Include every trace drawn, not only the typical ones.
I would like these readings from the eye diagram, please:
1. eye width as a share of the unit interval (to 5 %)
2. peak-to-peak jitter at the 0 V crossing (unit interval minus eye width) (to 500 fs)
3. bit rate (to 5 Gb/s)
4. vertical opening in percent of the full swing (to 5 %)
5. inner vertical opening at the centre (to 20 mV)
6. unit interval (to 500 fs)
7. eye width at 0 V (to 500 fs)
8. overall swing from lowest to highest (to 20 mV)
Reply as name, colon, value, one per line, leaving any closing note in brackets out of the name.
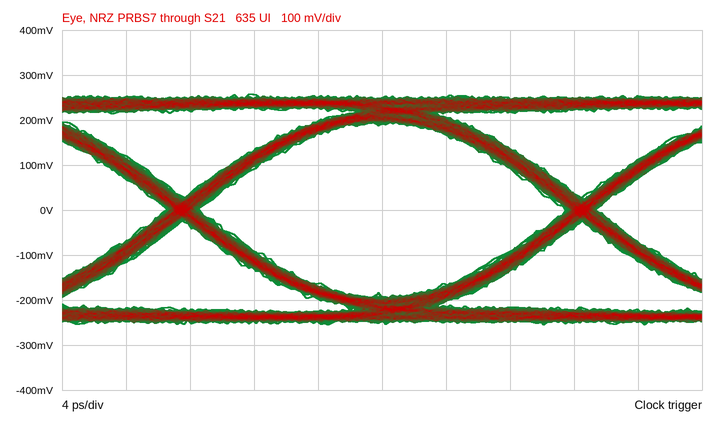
eye width as a share of the unit interval: 90 %
peak-to-peak jitter at the 0 V crossing (unit interval minus eye width): 2.0 ps
bit rate: 40 Gb/s
vertical opening in percent of the full swing: 75 %
inner vertical opening at the centre: 380 mV
unit interval: 25.0 ps
eye width at 0 V: 23.0 ps
overall swing from lowest to highest: 520 mV
